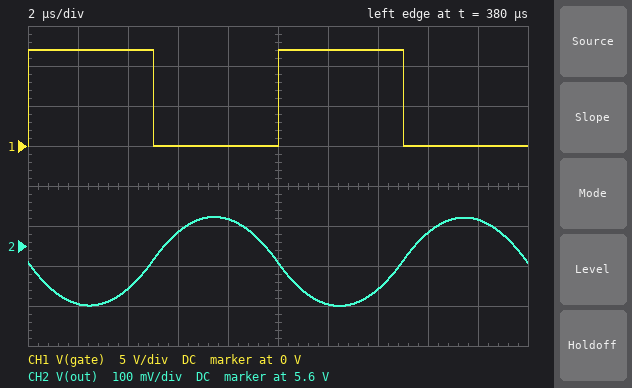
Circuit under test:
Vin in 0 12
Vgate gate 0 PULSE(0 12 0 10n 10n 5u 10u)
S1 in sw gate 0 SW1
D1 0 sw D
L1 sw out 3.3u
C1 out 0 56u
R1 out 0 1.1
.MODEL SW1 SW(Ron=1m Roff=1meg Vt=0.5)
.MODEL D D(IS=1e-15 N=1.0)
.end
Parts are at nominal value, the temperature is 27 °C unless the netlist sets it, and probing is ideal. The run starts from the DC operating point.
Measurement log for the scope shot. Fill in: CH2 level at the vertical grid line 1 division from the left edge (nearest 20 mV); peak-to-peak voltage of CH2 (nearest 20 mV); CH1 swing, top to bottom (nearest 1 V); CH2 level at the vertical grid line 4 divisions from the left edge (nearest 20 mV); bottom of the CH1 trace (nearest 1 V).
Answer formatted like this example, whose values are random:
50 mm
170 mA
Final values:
5.46 V
220 mV
12 V
5.66 V
0 V
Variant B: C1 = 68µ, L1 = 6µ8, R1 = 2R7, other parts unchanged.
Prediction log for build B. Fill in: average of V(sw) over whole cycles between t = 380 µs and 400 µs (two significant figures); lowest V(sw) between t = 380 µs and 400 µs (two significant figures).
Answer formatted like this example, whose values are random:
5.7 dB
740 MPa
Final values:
5.9 V
-930 mV
